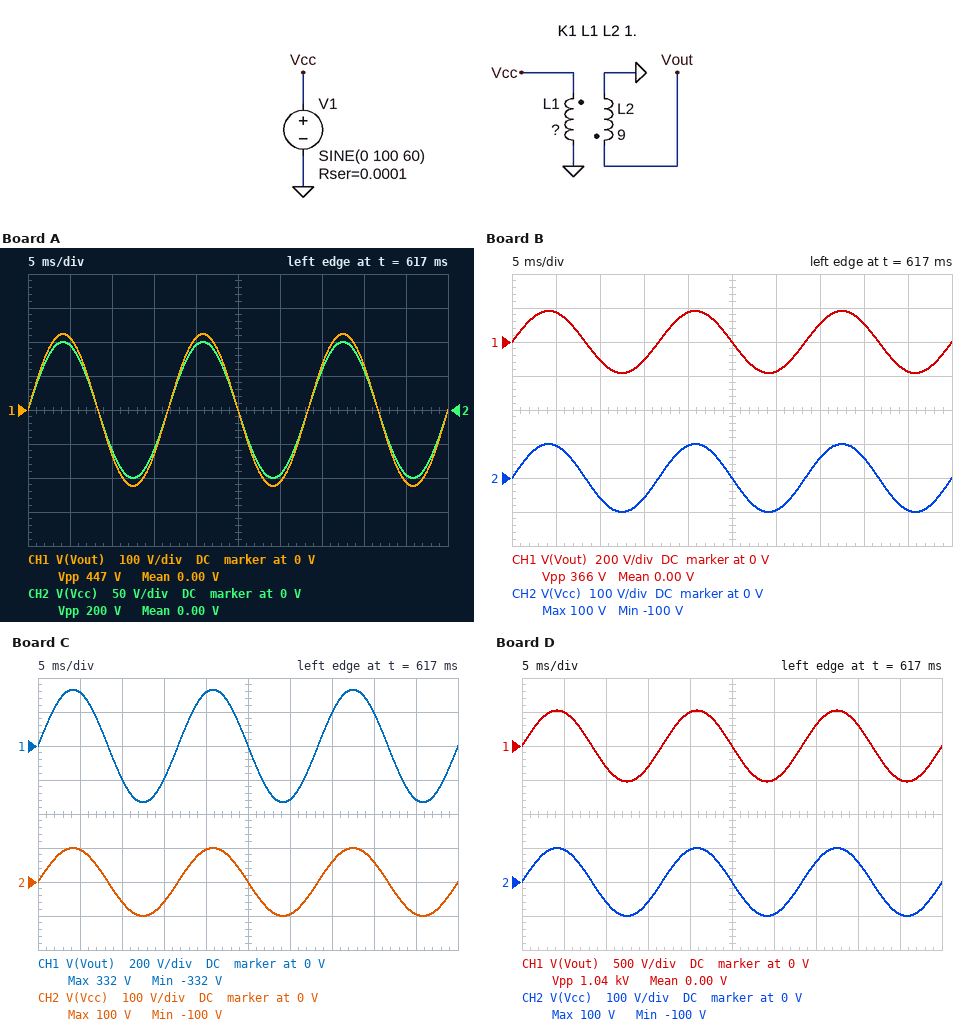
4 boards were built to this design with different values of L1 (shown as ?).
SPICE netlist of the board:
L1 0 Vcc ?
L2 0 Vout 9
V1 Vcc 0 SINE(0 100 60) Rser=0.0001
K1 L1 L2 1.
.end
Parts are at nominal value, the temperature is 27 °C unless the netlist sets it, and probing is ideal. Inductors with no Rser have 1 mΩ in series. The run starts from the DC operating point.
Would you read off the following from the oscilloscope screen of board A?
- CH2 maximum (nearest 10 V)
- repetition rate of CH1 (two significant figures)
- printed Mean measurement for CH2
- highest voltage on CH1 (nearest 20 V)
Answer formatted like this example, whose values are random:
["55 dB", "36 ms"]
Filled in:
["100 V", "60 Hz", "0.00 V", "220 V"]
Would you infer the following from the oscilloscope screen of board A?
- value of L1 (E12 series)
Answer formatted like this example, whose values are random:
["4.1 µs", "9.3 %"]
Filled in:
["1.8 H"]
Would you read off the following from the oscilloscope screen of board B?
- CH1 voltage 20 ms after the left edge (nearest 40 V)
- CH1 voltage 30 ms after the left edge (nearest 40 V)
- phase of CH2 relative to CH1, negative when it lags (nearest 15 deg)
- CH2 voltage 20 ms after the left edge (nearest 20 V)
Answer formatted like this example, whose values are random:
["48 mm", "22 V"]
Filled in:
["160 V", "-160 V", "0 deg", "100 V"]
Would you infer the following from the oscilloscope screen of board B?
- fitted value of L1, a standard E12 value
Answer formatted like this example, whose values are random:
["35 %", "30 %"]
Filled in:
["2.7 H"]
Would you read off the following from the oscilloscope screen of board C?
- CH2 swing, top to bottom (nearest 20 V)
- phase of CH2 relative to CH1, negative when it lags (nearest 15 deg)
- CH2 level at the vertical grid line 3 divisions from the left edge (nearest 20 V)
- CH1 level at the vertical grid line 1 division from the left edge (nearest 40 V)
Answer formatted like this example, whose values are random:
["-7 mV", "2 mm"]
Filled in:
["200 V", "0 deg", "-60 V", "320 V"]
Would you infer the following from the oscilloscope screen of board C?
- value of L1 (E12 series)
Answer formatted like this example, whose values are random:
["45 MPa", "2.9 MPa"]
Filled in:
["820 mH"]
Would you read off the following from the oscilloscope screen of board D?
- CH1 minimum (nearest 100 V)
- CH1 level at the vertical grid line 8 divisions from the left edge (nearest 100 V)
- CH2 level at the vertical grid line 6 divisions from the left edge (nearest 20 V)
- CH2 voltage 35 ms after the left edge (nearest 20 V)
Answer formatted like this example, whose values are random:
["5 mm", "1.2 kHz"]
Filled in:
["-500 V", "300 V", "-100 V", "60 V"]
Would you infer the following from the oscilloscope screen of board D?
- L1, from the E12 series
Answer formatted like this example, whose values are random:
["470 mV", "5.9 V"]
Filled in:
["330 mH"]
